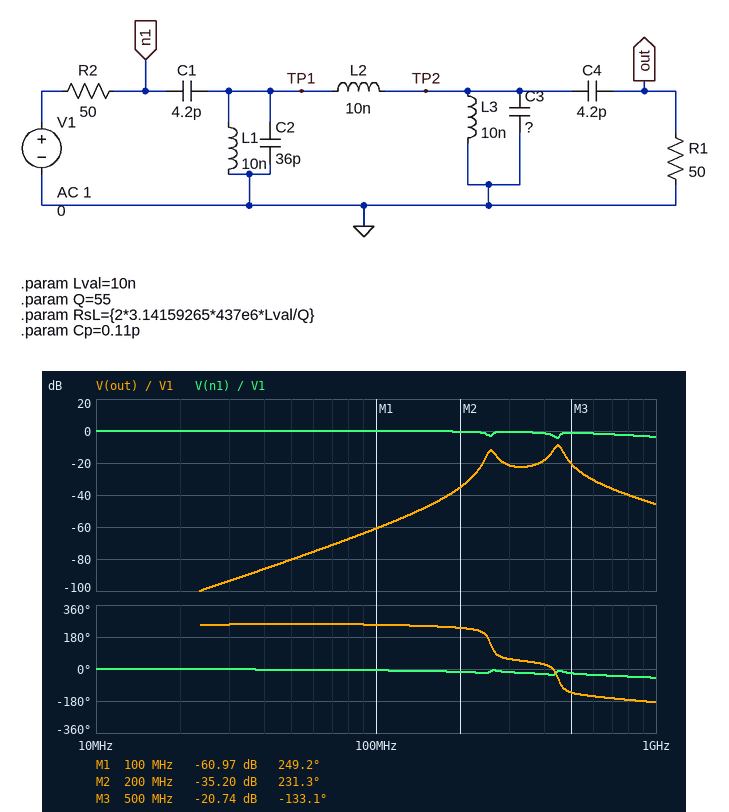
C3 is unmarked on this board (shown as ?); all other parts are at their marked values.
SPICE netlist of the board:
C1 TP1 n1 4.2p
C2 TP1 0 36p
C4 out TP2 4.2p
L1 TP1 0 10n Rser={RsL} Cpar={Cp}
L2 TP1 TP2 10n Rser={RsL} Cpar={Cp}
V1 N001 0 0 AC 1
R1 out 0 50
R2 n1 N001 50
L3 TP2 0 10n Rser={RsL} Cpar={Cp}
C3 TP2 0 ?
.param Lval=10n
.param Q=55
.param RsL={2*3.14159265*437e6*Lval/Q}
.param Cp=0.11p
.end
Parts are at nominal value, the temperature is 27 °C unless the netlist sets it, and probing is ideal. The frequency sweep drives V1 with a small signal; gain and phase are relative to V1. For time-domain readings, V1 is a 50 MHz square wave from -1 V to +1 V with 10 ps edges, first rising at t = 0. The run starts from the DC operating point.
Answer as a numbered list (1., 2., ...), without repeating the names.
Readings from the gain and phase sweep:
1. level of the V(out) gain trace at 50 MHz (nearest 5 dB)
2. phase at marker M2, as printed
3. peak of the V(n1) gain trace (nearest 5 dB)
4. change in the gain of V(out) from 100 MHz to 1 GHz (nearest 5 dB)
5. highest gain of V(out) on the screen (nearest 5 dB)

1. -80 dB
2. 231.3 deg
3. 0 dB
4. 15 dB
5. -10 dB
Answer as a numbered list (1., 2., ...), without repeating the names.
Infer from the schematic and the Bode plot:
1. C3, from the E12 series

1. 33 pF
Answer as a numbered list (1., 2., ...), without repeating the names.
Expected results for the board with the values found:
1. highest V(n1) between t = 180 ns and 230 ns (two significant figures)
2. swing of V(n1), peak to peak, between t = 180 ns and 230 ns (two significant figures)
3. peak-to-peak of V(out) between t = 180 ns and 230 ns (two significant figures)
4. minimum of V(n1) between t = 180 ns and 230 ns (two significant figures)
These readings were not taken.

1. 1.1 V
2. 2.2 V
3. 230 mV
4. -1.1 V
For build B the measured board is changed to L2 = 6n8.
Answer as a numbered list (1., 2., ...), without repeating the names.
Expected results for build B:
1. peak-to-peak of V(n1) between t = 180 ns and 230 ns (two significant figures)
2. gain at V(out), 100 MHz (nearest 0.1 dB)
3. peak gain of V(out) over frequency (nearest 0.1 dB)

1. 2.1 V
2. -60.1 dB
3. -9.0 dB
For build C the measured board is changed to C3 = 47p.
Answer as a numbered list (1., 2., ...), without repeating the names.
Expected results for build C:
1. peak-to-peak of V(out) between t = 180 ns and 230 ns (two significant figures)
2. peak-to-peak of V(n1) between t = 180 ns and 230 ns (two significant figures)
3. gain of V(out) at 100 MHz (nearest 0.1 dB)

1. 100 mV
2. 2.1 V
3. -60.6 dB
